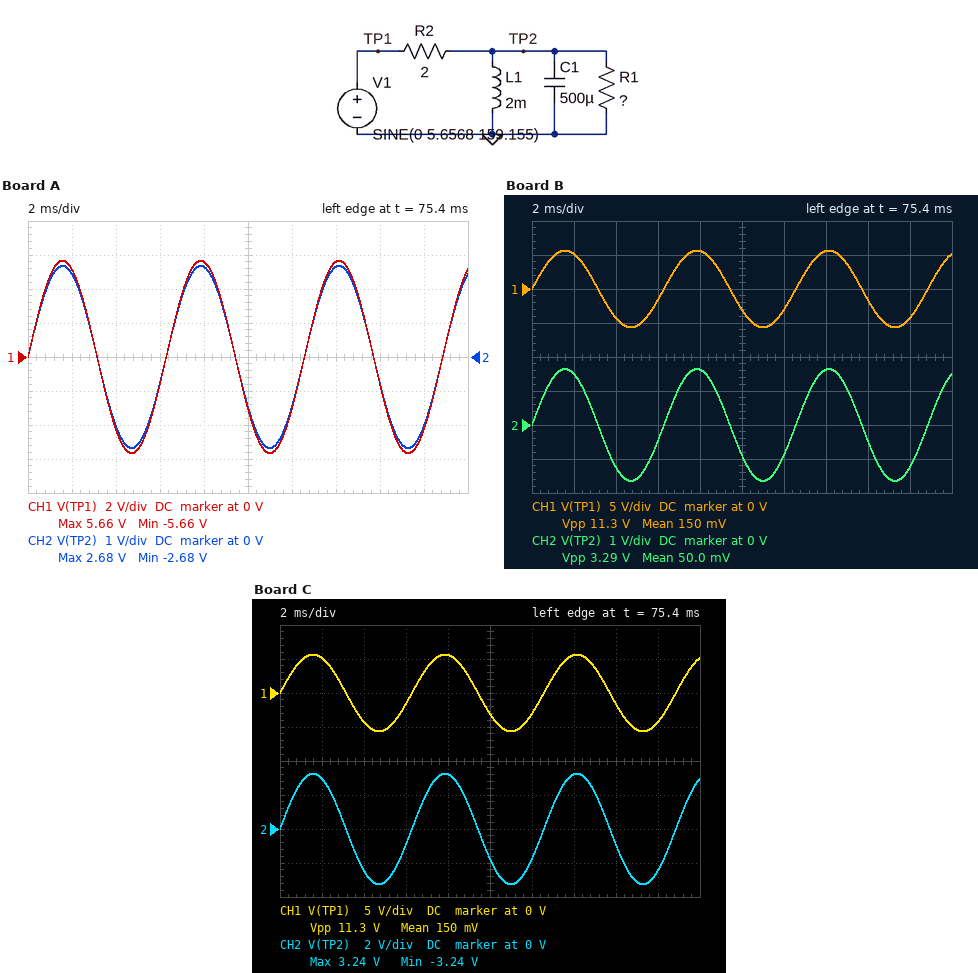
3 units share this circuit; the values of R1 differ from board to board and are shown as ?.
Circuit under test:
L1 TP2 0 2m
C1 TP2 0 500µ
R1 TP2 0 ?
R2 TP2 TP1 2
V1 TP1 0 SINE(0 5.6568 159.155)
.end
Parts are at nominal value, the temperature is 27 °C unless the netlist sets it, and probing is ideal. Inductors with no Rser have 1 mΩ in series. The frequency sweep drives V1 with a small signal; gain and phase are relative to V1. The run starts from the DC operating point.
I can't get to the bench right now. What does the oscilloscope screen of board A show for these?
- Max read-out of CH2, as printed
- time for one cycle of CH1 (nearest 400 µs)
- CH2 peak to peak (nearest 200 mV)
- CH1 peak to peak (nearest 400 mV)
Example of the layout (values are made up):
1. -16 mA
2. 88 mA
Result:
1. 2.68 V
2. 6.4 ms
3. 5.4 V
4. 11.2 V
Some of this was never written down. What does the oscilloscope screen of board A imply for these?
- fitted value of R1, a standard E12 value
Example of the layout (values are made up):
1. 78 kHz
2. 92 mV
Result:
1. 1.8 Ω
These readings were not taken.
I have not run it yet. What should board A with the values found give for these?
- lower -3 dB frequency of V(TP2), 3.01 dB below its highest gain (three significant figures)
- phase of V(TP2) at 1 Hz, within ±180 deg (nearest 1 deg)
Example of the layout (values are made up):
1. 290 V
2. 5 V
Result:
1. 63.5 Hz
2. 85 deg
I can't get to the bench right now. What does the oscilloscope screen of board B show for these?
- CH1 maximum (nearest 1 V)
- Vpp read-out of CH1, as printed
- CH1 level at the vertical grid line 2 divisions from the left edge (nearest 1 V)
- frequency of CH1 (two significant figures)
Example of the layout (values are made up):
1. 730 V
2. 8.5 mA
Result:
1. 6 V
2. 11.3 V
3. -4 V
4. 160 Hz
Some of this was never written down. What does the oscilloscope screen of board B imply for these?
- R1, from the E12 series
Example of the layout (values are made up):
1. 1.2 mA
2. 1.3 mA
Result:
1. 0.82 Ω
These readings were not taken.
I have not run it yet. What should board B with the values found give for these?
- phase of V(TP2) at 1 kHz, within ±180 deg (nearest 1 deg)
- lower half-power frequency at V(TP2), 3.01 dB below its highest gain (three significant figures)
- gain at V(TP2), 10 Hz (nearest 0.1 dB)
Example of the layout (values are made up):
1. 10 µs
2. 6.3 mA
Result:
1. -61 deg
2. 43.0 Hz
3. -24.2 dB
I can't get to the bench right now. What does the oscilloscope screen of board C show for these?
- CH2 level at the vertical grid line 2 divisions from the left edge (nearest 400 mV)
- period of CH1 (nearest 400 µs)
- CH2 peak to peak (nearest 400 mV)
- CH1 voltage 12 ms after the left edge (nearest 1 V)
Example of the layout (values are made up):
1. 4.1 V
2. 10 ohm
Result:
1. -2.4 V
2. 6.4 ms
3. 6.4 V
4. -3 V
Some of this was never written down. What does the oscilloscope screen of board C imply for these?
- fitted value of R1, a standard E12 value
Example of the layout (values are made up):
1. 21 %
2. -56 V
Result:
1. 2.7 Ω
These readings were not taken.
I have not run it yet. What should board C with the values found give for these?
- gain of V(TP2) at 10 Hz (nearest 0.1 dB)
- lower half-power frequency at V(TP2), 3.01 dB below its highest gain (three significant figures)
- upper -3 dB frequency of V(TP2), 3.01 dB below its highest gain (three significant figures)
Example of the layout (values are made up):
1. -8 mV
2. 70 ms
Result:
1. -24.1 dB
2. 72.5 Hz
3. 350 Hz
